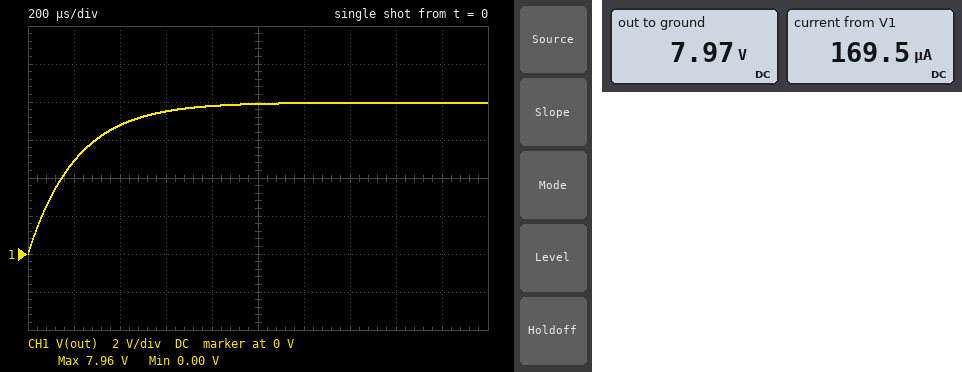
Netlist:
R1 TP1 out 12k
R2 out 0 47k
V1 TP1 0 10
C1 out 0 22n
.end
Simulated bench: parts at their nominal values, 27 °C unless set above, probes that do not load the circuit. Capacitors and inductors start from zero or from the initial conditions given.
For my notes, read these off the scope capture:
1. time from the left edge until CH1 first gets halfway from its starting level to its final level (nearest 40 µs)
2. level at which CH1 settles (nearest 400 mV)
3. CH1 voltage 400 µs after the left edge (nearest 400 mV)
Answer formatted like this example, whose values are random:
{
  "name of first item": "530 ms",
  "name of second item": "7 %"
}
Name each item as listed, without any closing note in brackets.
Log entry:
{
  "time from the left edge until CH1 first gets halfway from its starting level to its final level": "160 µs",
  "level at which CH1 settles": "8.0 V",
  "CH1 voltage 400 µs after the left edge": "6.8 V"
}
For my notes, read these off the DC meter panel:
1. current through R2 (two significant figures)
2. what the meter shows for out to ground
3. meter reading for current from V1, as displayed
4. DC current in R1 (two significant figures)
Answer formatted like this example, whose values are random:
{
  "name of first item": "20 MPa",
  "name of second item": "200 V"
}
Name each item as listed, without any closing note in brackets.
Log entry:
{
  "current through R2": "170 µA",
  "what the meter shows for out to ground": "7.97 V",
  "meter reading for current from V1, as displayed": "169.5 µA",
  "DC current in R1": "170 µA"
}
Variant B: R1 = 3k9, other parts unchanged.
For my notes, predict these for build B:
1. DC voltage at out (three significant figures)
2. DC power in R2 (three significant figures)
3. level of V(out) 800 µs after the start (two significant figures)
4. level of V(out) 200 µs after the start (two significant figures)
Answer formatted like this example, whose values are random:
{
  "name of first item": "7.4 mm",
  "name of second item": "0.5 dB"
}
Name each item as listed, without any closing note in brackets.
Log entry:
{
  "DC voltage at out": "9.23 V",
  "DC power in R2": "1.81 mW",
  "level of V(out) 800 µs after the start": "9.2 V",
  "level of V(out) 200 µs after the start": "8.5 V"
}
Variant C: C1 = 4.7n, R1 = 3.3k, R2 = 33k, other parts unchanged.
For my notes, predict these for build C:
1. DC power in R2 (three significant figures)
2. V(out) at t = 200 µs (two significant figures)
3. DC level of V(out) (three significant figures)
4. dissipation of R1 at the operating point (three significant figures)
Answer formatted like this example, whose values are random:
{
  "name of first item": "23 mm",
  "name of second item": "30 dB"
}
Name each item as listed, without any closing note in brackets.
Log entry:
{
  "DC power in R2": "2.50 mW",
  "V(out) at t = 200 µs": "9.1 V",
  "DC level of V(out)": "9.09 V",
  "dissipation of R1 at the operating point": "250 µW"
}
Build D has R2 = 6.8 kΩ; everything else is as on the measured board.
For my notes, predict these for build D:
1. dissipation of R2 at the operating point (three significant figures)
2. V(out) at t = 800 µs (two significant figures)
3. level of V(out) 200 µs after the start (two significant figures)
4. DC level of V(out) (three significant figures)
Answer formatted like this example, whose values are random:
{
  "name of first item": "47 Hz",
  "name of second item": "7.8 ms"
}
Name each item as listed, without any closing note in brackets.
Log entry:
{
  "dissipation of R2 at the operating point": "1.92 mW",
  "V(out) at t = 800 µs": "3.6 V",
  "level of V(out) 200 µs after the start": "3.2 V",
  "DC level of V(out)": "3.62 V"
}
